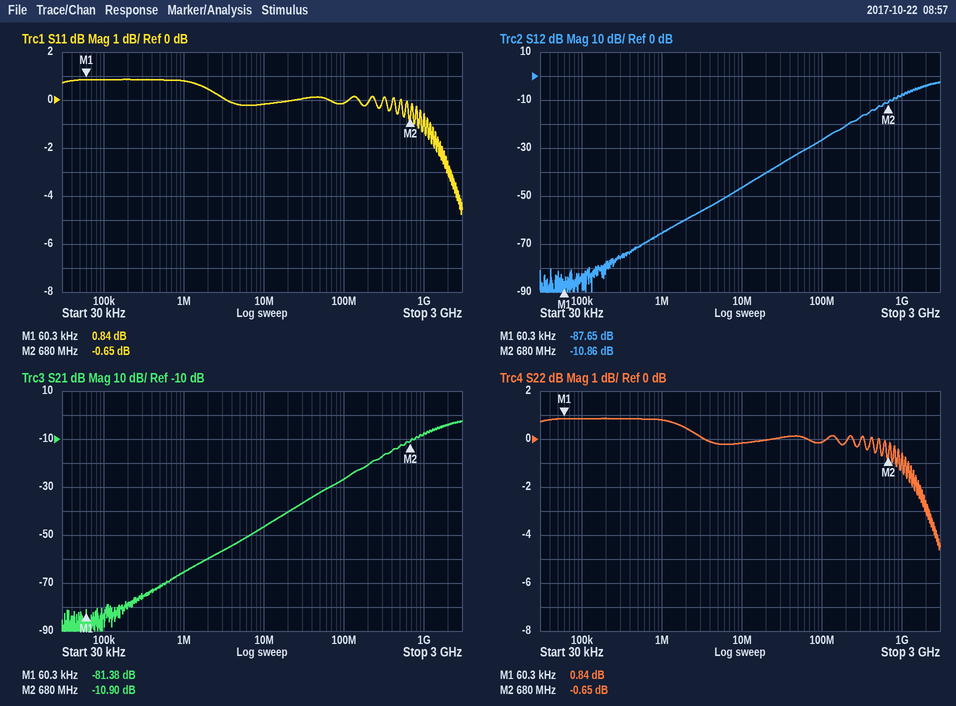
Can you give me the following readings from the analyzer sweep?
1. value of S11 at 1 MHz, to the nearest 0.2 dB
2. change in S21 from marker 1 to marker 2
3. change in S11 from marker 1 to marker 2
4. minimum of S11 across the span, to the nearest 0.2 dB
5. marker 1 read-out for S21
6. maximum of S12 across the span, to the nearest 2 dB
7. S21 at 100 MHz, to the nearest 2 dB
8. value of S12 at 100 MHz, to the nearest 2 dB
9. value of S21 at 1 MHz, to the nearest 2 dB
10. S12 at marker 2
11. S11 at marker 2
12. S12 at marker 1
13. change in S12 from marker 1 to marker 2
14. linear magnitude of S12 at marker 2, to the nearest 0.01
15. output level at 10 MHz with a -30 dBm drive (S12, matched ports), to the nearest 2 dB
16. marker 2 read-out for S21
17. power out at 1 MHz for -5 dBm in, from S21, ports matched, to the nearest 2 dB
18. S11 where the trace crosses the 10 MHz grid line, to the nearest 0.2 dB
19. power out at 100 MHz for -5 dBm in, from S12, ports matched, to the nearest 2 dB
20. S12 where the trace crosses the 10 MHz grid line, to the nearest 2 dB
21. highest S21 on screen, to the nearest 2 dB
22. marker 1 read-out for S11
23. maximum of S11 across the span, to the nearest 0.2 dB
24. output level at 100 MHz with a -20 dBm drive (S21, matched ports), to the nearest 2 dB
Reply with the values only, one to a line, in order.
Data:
0.8 dB
70.48 dB
-1.49 dB
-4.8 dB
-81.38 dB
-2 dB
-26 dB
-26 dB
-66 dB
-10.86 dB
-0.65 dB
-87.65 dB
76.79 dB
0.29
-76 dBm
-10.90 dB
-70 dBm
-0.2 dB
-32 dBm
-46 dB
-2 dB
0.84 dB
0.8 dB
-46 dBm
